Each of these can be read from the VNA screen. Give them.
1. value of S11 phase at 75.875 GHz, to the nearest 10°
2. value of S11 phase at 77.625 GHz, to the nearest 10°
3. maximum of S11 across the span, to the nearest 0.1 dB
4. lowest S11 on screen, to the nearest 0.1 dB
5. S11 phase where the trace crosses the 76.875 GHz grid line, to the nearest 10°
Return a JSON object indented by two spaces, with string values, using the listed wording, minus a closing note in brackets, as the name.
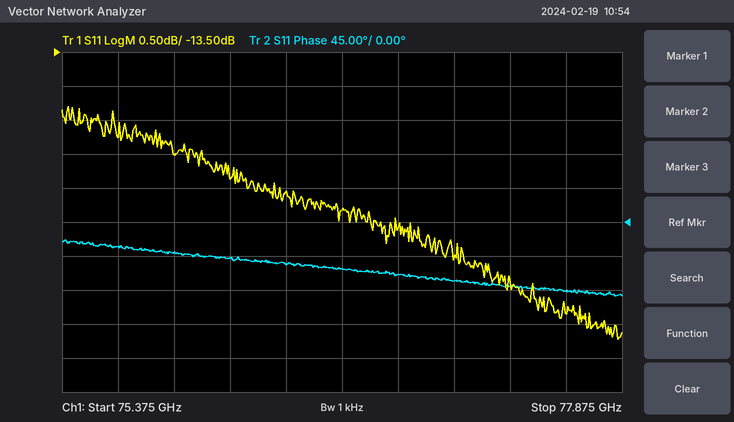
{
  "value of S11 phase at 75.875 GHz, to the nearest 10°": "-40°",
  "value of S11 phase at 77.625 GHz, to the nearest 10°": "-90°",
  "maximum of S11 across the span, to the nearest 0.1 dB": "-14.3 dB",
  "lowest S11 on screen, to the nearest 0.1 dB": "-17.7 dB",
  "S11 phase where the trace crosses the 76.875 GHz grid line, to the nearest 10°": "-70°"
}
